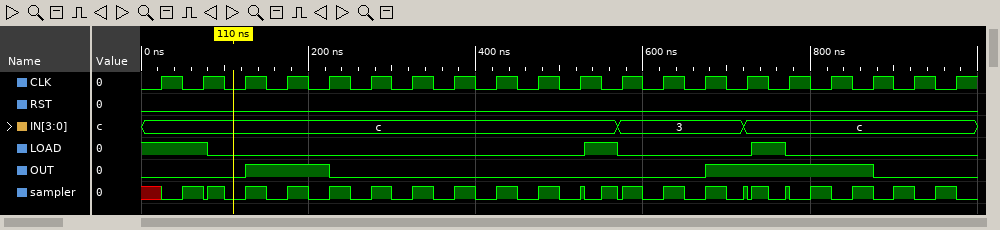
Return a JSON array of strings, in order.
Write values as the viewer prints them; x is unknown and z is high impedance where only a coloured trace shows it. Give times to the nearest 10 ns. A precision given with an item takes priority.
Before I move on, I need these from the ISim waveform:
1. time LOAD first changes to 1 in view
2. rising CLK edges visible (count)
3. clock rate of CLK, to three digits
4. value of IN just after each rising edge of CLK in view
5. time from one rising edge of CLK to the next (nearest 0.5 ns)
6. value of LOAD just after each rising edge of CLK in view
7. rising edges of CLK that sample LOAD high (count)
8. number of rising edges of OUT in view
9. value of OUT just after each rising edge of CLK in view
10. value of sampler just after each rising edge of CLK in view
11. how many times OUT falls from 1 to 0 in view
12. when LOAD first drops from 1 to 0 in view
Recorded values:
["530 ns", "20", "20.0 MHz", "c, c, c, c, c, c, c, c, c, c, c, 3, 3, 3, c, c, c, c, c, c", "50 ns", "1 1 0 0 0 0 0 0 0 0 0 0 0 0 0 0 0 0 0 0", "2", "2", "0 0 1 1 0 0 0 0 0 0 0 0 0 1 1 1 1 0 0 0", "0 0 1 1 1 1 1 1 1 1 1 1 1 1 0 0 0 0 0 0", "2", "80 ns"]
